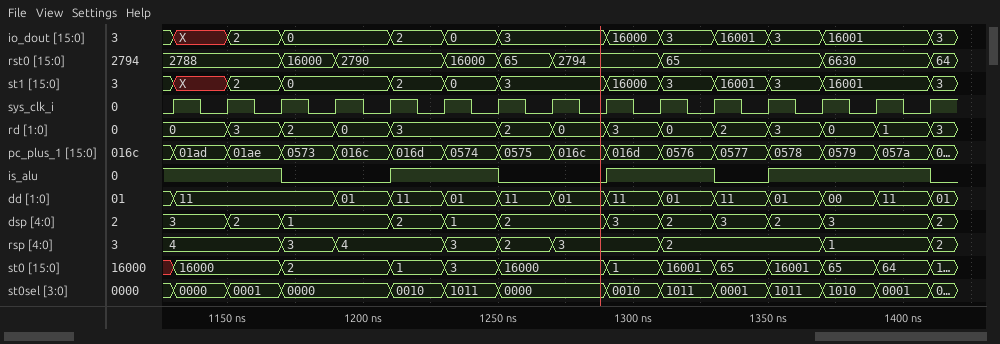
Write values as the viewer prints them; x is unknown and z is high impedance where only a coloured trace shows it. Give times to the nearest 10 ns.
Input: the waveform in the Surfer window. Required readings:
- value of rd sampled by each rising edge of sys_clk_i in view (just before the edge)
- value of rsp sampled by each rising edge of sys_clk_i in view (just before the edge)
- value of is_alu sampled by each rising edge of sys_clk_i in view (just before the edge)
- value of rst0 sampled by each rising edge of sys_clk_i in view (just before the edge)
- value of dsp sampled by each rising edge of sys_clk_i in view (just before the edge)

0, 0, 3, 2, 0, 3, 3, 2, 0, 3, 0, 2, 3, 0, 1
4, 4, 4, 3, 4, 4, 3, 2, 3, 3, 2, 2, 2, 1, 1
1 1 1 0 0 1 1 0 0 1 1 0 1 1 1
2788, 2788, 2788, 16000, 2790, 2790, 16000, 65, 2794, 2794, 65, 65, 65, 6630, 6630
3, 3, 2, 1, 1, 2, 1, 2, 2, 3, 2, 3, 2, 3, 3
